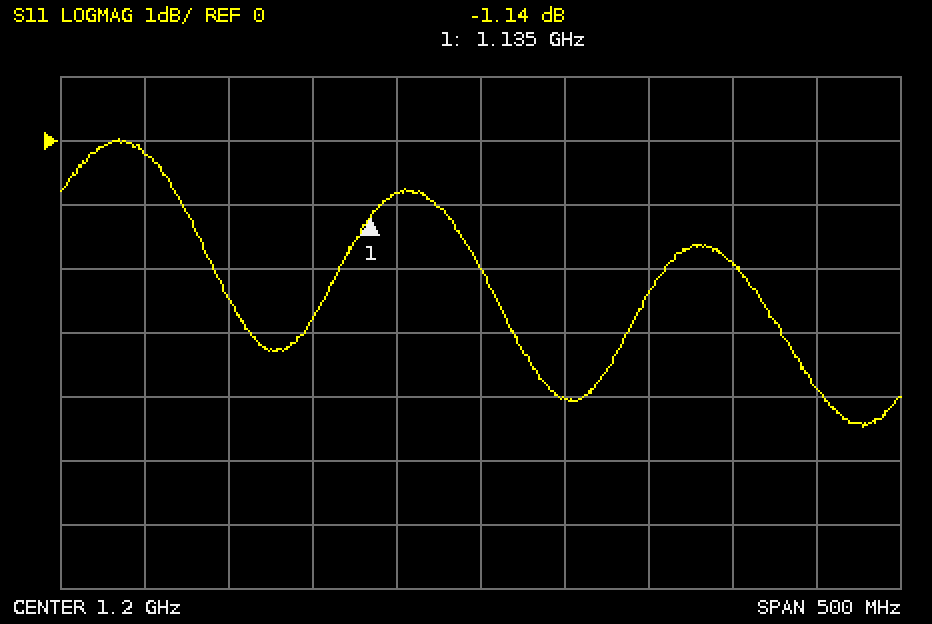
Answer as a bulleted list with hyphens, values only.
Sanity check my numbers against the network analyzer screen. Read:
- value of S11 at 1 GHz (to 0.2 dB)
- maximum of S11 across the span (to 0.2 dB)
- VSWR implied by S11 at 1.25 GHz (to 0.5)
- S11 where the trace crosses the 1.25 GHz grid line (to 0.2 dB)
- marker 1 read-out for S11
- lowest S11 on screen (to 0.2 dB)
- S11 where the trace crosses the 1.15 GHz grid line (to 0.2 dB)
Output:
- -0.2 dB
- 0.0 dB
- 4.5
- -4.0 dB
- -1.14 dB
- -4.4 dB
- -0.8 dB
